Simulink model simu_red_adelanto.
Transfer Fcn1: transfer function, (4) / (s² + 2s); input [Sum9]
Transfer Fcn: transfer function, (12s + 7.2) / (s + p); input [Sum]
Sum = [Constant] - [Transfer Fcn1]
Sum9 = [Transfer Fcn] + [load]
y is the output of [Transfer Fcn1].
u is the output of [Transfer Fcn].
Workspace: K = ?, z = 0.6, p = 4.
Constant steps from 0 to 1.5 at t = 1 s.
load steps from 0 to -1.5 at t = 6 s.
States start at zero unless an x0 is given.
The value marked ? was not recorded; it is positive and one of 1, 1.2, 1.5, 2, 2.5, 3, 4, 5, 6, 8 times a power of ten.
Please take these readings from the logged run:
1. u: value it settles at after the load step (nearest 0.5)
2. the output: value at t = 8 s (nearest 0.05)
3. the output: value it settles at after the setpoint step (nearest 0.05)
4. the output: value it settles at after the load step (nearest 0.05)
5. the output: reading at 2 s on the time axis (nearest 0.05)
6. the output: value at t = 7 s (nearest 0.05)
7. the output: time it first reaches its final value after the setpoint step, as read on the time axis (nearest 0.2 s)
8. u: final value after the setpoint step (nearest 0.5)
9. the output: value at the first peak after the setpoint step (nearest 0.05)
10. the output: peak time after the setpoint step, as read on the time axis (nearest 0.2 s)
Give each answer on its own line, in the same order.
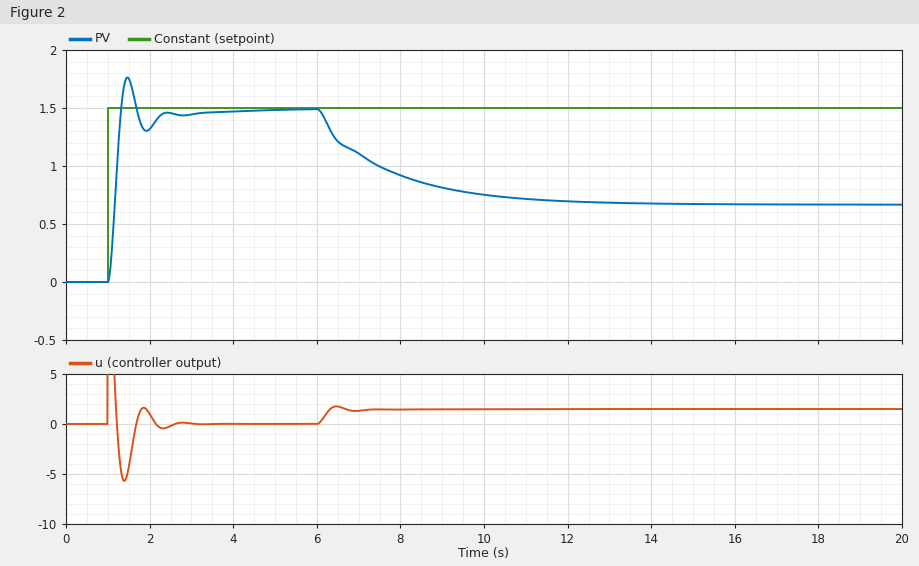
1.5
0.90
1.50
0.65
1.30
1.10
1.4 s
0.0
1.75
1.4 s
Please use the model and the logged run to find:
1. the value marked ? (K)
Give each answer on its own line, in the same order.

12
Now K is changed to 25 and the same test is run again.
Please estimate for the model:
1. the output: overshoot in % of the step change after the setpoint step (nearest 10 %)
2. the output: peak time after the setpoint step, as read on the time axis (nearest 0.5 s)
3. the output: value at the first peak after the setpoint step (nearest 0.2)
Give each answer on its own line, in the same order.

40 %
1.5 s
2.0
